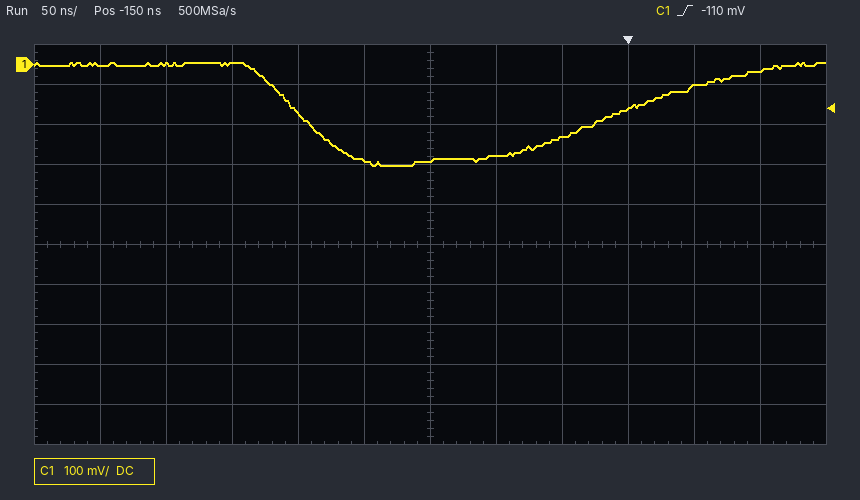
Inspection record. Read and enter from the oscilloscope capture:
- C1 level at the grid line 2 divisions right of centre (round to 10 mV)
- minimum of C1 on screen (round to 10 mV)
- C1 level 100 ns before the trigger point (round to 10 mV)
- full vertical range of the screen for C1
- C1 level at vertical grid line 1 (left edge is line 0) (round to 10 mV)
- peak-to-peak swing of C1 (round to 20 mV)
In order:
-180 mV
-250 mV
-230 mV
1 V
0 mV
260 mV
